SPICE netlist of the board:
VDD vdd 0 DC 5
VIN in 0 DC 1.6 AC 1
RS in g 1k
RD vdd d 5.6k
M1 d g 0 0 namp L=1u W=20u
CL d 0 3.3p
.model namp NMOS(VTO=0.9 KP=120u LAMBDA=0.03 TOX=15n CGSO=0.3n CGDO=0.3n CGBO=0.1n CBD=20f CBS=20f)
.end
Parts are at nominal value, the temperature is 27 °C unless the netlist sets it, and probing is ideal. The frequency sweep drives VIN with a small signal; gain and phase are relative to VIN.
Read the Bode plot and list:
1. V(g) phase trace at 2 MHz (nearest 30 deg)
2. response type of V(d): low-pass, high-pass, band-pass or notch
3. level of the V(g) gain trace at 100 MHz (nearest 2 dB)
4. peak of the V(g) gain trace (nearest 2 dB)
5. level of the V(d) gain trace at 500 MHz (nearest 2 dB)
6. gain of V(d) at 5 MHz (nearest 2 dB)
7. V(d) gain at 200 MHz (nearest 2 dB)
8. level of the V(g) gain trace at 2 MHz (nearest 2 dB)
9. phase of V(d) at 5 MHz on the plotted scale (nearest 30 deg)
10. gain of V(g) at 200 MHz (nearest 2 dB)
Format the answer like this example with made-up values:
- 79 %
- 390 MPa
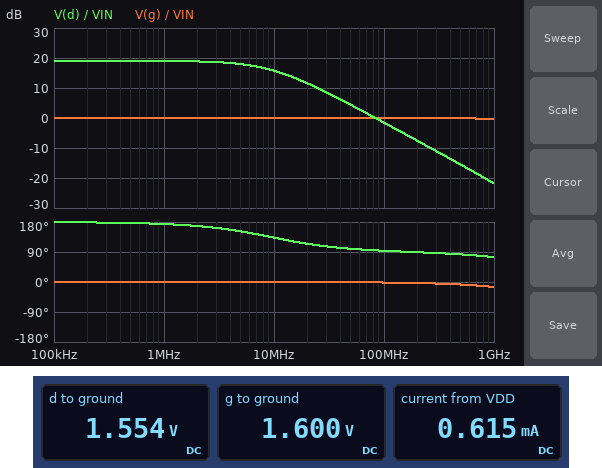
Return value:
- 0 deg
- low-pass
- 0 dB
- 0 dB
- -16 dB
- 18 dB
- -8 dB
- 0 dB
- 150 deg
- 0 dB
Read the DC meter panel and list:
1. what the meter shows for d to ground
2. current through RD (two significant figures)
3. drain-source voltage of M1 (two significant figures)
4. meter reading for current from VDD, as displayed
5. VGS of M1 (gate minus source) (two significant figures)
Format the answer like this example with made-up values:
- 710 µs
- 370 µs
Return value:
- 1.554 V
- 620 µA
- 1.6 V
- 0.615 mA
- 1.6 V
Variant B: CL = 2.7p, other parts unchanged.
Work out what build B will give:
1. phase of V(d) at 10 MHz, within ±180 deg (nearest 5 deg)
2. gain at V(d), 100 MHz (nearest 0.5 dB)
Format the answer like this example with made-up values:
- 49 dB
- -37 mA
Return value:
- 140 deg
- 0 dB
